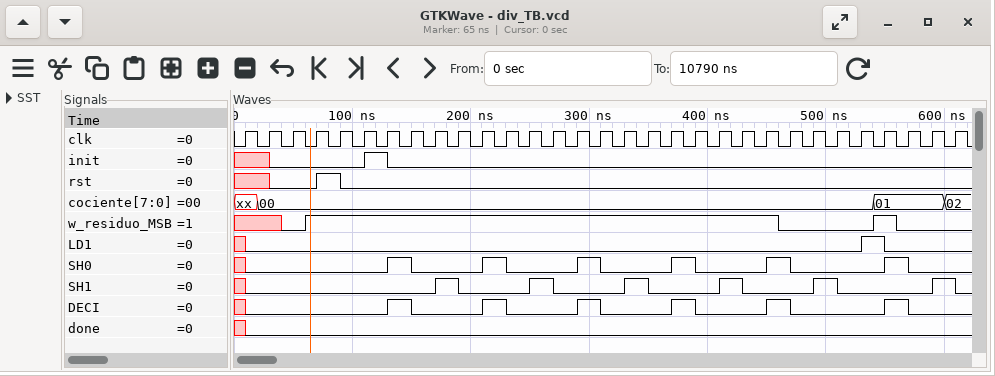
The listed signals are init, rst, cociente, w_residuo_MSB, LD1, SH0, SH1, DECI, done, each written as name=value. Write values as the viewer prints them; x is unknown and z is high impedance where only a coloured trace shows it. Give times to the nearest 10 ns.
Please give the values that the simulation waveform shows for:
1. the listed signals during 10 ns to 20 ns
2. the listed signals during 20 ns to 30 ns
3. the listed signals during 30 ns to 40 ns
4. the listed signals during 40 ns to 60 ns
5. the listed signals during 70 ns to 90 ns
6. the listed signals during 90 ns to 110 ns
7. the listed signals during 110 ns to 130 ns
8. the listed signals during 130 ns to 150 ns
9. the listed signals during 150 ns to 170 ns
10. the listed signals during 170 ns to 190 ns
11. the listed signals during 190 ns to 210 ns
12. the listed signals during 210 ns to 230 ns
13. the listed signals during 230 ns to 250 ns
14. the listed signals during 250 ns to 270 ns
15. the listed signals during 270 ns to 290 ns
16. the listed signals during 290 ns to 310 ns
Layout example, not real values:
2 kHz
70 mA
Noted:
init=x, rst=x, cociente=xx, w_residuo_MSB=x, LD1=0, SH0=0, SH1=0, DECI=0, done=0
init=x, rst=x, cociente=00, w_residuo_MSB=x, LD1=0, SH0=0, SH1=0, DECI=0, done=0
init=0, rst=0, cociente=00, w_residuo_MSB=x, LD1=0, SH0=0, SH1=0, DECI=0, done=0
init=0, rst=0, cociente=00, w_residuo_MSB=0, LD1=0, SH0=0, SH1=0, DECI=0, done=0
init=0, rst=1, cociente=00, w_residuo_MSB=1, LD1=0, SH0=0, SH1=0, DECI=0, done=0
init=0, rst=0, cociente=00, w_residuo_MSB=1, LD1=0, SH0=0, SH1=0, DECI=0, done=0
init=1, rst=0, cociente=00, w_residuo_MSB=1, LD1=0, SH0=0, SH1=0, DECI=0, done=0
init=0, rst=0, cociente=00, w_residuo_MSB=1, LD1=0, SH0=1, SH1=0, DECI=1, done=0
init=0, rst=0, cociente=00, w_residuo_MSB=1, LD1=0, SH0=0, SH1=0, DECI=0, done=0
init=0, rst=0, cociente=00, w_residuo_MSB=1, LD1=0, SH0=0, SH1=1, DECI=0, done=0
init=0, rst=0, cociente=00, w_residuo_MSB=1, LD1=0, SH0=0, SH1=0, DECI=0, done=0
init=0, rst=0, cociente=00, w_residuo_MSB=1, LD1=0, SH0=1, SH1=0, DECI=1, done=0
init=0, rst=0, cociente=00, w_residuo_MSB=1, LD1=0, SH0=0, SH1=0, DECI=0, done=0
init=0, rst=0, cociente=00, w_residuo_MSB=1, LD1=0, SH0=0, SH1=1, DECI=0, done=0
init=0, rst=0, cociente=00, w_residuo_MSB=1, LD1=0, SH0=0, SH1=0, DECI=0, done=0
init=0, rst=0, cociente=00, w_residuo_MSB=1, LD1=0, SH0=1, SH1=0, DECI=1, done=0
